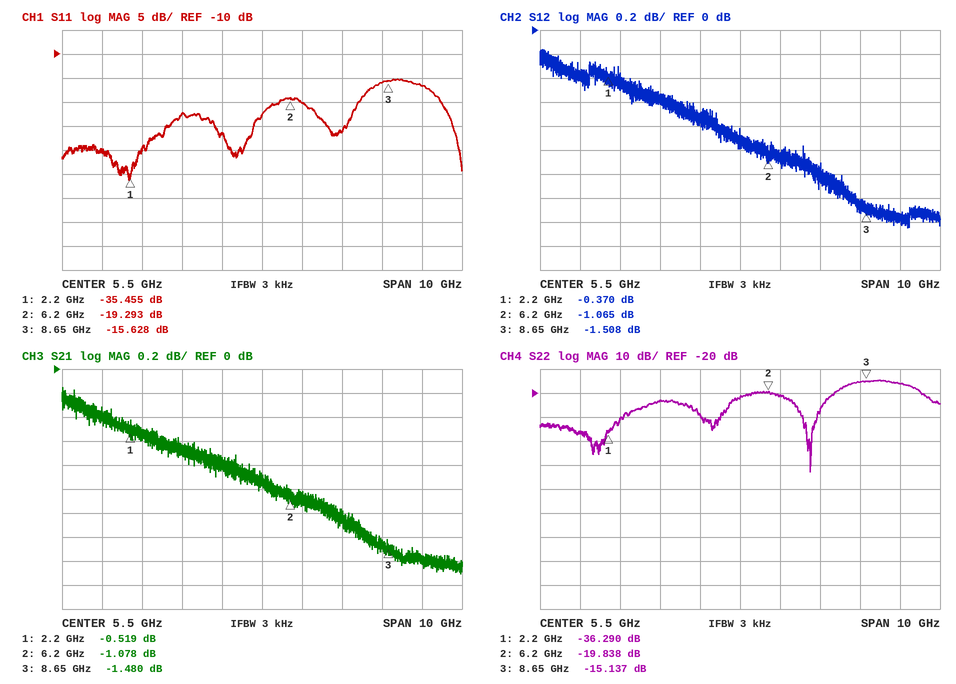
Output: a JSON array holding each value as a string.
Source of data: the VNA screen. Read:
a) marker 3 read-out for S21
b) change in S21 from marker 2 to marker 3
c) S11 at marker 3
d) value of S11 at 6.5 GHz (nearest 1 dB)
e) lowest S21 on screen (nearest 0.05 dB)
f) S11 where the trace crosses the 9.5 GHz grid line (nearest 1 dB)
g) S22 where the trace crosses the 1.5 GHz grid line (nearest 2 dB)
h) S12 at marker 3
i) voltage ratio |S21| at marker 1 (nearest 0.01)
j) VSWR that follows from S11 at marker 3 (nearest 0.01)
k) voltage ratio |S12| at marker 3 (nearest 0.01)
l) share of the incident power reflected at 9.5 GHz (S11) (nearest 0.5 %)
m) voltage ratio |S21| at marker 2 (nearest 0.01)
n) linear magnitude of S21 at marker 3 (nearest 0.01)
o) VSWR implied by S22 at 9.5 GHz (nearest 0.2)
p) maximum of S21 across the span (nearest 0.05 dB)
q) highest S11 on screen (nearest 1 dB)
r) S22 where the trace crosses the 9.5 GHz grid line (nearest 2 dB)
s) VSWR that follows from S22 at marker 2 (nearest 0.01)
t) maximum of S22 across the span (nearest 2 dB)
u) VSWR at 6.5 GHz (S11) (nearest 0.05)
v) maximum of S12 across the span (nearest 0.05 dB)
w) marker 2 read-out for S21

["-1.480 dB", "-0.402 dB", "-15.628 dB", "-20 dB", "-1.70 dB", "-17 dB", "-36 dB", "-1.508 dB", "0.94", "1.40", "0.84", "2.0 %", "0.88", "0.84", "1.4", "-0.15 dB", "-15 dB", "-16 dB", "1.23", "-14 dB", "1.20", "-0.15 dB", "-1.078 dB"]
